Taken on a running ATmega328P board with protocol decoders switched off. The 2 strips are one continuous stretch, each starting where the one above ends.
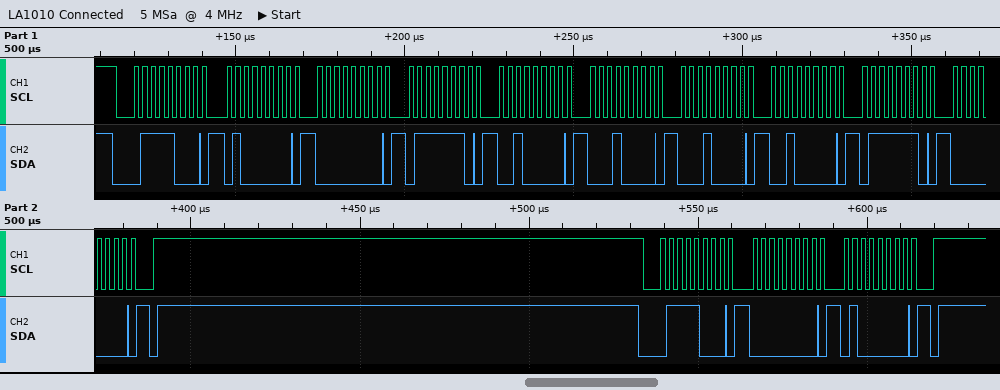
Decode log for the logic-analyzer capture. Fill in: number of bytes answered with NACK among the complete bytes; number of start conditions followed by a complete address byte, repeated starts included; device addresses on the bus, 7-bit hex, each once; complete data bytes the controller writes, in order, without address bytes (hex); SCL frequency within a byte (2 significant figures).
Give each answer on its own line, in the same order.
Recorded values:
0
2
0x3C
40 00 7E 20 10 10 20 7E 00 00 40
400 kHz
